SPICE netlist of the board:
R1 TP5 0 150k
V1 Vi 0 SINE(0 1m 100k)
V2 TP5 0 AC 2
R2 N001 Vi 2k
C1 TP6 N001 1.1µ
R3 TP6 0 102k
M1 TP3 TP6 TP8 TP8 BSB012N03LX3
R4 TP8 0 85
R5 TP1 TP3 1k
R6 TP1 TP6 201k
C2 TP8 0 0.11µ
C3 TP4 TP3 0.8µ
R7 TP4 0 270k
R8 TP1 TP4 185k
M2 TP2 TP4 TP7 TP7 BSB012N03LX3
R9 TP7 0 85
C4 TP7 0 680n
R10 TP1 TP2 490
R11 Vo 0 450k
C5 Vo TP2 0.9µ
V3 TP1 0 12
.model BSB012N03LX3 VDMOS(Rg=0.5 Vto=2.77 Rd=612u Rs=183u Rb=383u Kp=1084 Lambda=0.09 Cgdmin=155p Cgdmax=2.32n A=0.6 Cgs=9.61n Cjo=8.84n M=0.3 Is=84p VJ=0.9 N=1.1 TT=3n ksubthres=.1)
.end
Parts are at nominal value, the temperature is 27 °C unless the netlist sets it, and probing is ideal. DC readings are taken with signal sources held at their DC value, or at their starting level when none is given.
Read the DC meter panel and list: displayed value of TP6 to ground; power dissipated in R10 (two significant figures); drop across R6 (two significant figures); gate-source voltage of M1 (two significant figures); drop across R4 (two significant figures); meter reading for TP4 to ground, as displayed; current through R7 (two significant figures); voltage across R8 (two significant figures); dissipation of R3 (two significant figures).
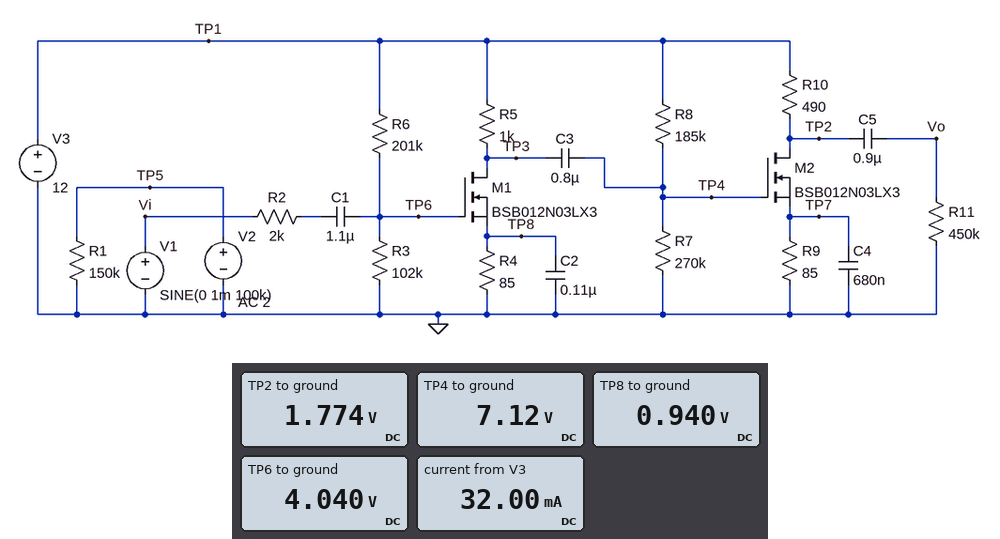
4.040 V
210 mW
8.0 V
3.1 V
940 mV
7.12 V
26 µA
4.9 V
160 µW
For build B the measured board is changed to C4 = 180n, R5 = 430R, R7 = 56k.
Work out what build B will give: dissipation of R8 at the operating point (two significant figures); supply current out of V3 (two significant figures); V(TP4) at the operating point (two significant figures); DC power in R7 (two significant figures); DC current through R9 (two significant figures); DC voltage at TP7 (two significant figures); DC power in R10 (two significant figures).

460 µW
23 mA
2.8 V
140 µW
4.7 mA
400 mV
11 mW
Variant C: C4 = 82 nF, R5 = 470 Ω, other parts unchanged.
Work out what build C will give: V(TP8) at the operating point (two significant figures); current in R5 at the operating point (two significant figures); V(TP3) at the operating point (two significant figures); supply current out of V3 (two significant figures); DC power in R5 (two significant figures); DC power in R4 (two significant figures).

1.6 V
18 mA
3.4 V
39 mA
160 mW
29 mW
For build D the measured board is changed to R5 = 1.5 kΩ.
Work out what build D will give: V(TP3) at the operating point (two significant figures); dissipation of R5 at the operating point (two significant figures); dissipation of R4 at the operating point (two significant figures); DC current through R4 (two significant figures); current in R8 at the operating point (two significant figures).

640 mV
86 mW
4.9 mW
7.6 mA
26 µA
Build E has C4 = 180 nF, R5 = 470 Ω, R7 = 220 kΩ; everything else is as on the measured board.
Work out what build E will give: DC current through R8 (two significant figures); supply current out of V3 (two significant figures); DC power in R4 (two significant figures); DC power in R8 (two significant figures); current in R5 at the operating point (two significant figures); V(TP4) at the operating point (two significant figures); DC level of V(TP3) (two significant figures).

30 µA
39 mA
29 mW
160 µW
18 mA
6.5 V
3.4 V
